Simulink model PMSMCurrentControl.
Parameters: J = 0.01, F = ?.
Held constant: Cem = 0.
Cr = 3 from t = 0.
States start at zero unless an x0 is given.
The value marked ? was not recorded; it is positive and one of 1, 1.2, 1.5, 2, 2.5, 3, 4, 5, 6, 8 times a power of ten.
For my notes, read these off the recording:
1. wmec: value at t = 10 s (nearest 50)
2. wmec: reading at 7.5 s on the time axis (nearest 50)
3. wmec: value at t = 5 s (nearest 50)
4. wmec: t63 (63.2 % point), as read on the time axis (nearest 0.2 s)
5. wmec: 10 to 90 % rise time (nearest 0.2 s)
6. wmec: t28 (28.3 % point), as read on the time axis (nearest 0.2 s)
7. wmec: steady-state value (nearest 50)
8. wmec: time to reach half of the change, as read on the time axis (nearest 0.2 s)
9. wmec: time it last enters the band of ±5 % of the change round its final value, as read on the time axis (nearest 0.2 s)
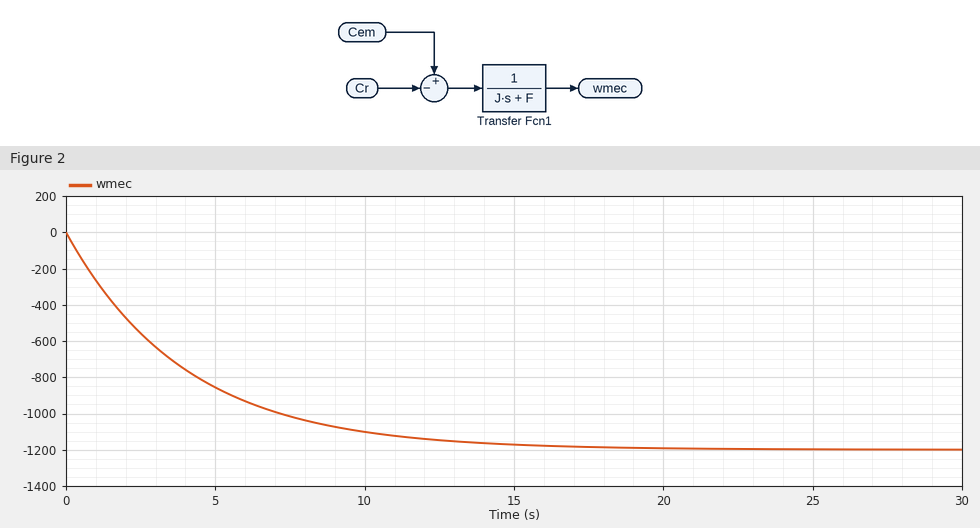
-1100
-1000
-850
4.0 s
8.8 s
1.4 s
-1200
2.8 s
12.0 s
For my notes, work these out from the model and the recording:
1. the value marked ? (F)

0.0025
